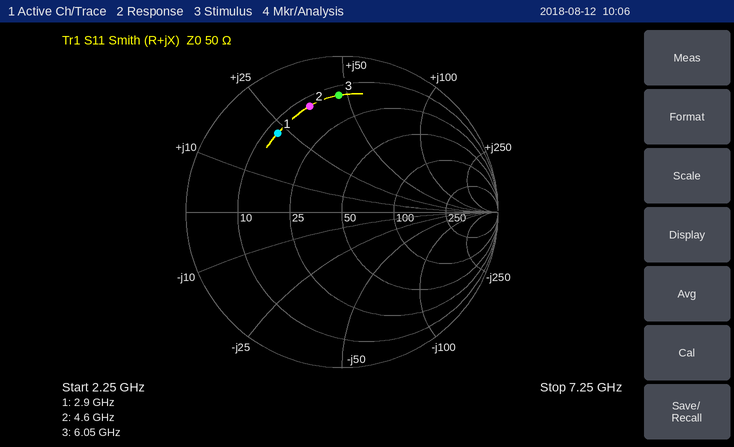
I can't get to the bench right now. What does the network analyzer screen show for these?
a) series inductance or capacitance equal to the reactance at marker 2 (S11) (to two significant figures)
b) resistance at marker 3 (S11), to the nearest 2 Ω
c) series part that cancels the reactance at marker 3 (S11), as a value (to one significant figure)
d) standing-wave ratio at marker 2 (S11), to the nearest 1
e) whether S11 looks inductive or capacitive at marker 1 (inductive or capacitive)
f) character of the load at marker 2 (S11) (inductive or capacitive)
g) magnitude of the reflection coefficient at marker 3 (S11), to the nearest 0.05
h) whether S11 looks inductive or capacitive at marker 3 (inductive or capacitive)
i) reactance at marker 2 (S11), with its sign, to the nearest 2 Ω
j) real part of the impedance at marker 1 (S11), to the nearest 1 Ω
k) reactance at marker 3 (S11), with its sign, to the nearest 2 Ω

1.2 nH
14 Ω
600 fF
6
inductive
inductive
0.75
inductive
+36 Ω
13 Ω
+46 Ω
